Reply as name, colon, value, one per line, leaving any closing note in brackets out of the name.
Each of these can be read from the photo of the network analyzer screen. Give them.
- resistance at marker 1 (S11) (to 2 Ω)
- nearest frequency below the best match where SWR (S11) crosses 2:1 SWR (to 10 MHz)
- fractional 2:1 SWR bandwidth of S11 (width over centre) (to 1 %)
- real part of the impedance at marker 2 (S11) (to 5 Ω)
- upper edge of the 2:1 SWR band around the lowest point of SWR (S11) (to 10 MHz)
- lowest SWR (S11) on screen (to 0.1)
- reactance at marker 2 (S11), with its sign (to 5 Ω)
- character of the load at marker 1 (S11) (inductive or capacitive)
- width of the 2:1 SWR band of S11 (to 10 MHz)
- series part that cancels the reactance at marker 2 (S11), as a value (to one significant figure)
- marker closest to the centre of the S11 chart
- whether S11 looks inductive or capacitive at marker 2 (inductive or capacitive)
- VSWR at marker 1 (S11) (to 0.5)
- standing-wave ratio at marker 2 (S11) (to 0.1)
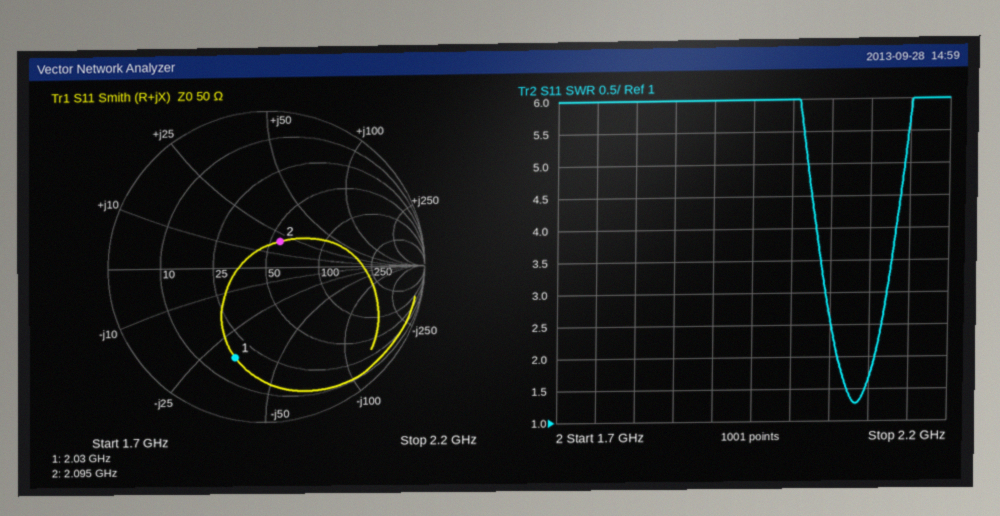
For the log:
resistance at marker 1 (S11): 18 Ω
nearest frequency below the best match where SWR (S11) crosses 2:1 SWR: 2.06 GHz
fractional 2:1 SWR bandwidth of S11 (width over centre): 2 %
real part of the impedance at marker 2 (S11): 55 Ω
upper edge of the 2:1 SWR band around the lowest point of SWR (S11): 2.11 GHz
lowest SWR (S11) on screen: 1.3
reactance at marker 2 (S11), with its sign: +20 Ω
character of the load at marker 1 (S11): capacitive
width of the 2:1 SWR band of S11: 50 MHz
series part that cancels the reactance at marker 2 (S11), as a value: 4 pF
marker closest to the centre of the S11 chart: marker 2
whether S11 looks inductive or capacitive at marker 2: inductive
VSWR at marker 1 (S11): 4.0
standing-wave ratio at marker 2 (S11): 1.5
